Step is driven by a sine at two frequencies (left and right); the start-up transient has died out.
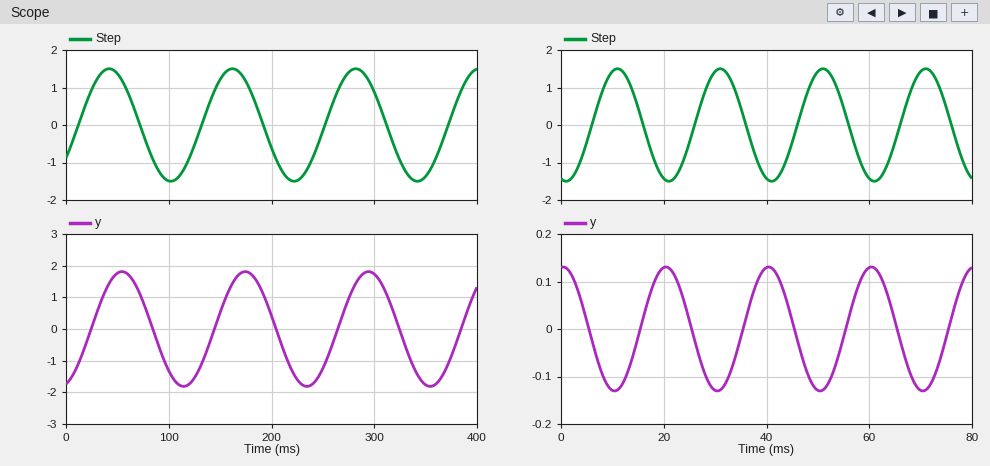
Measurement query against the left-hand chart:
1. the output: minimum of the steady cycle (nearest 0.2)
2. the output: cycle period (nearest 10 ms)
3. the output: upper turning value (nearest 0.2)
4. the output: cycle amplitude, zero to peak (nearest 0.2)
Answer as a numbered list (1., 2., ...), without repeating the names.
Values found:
1. -1.8
2. 120 ms
3. 1.8
4. 1.8
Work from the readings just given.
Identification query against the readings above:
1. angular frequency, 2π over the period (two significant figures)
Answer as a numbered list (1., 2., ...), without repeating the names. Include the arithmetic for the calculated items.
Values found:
1. 2π / 120 = 0.052 rad/ms
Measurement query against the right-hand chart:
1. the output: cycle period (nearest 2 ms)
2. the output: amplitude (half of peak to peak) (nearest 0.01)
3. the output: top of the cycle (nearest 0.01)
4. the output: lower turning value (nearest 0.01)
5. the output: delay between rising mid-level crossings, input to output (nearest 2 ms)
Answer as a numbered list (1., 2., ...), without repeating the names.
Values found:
1. 20 ms
2. 0.13
3. 0.13
4. -0.13
5. 10 ms
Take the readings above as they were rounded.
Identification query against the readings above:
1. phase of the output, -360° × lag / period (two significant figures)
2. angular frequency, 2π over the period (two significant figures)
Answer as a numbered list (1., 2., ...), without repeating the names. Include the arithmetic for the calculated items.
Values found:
1. -360 × 10 / 20 = -180°
2. 2π / 20 = 0.31 rad/ms
